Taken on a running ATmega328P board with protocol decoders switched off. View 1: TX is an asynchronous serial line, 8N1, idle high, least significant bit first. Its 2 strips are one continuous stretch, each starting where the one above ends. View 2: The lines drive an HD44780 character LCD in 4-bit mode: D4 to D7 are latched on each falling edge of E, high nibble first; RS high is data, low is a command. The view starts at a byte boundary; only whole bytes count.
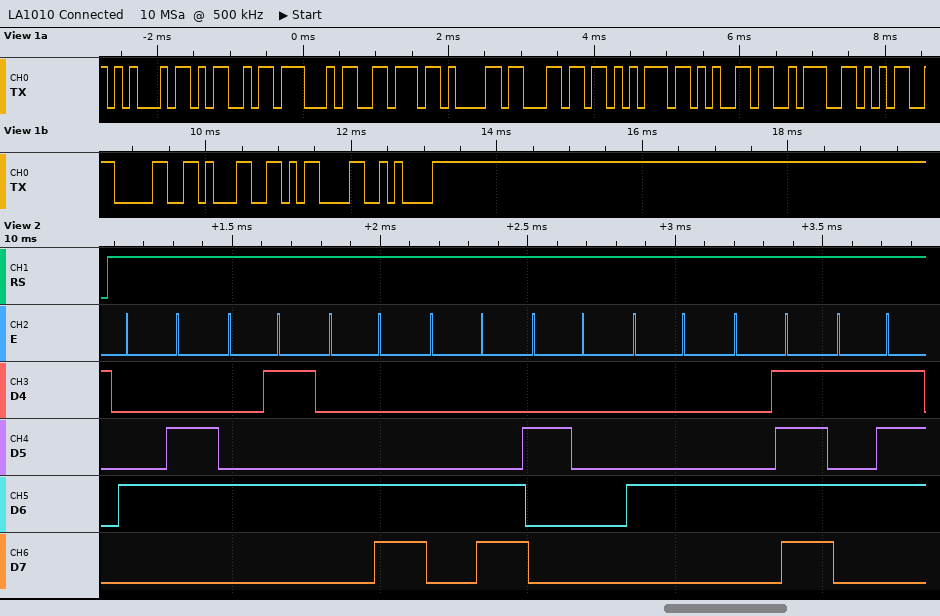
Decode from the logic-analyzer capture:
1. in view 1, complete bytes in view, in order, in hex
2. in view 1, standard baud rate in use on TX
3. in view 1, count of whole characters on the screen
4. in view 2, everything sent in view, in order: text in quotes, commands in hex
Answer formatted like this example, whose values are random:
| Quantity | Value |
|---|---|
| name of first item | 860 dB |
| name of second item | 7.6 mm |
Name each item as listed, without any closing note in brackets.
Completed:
| Quantity | Value |
|---|---|
| in view 1, complete bytes in view, in order, in hex | 45 4D 47 76 61 6C 75 65 3A 35 30 31 0D 0A |
| in view 1, standard baud rate in use on TX | 9600 baud |
| in view 1, count of whole characters on the screen | 14 |
| in view 2, everything sent in view, in order: text in quotes, commands in hex | "FELL DOW" |
